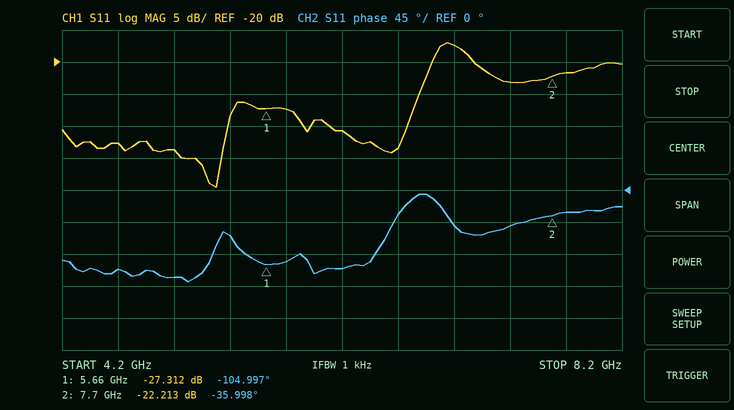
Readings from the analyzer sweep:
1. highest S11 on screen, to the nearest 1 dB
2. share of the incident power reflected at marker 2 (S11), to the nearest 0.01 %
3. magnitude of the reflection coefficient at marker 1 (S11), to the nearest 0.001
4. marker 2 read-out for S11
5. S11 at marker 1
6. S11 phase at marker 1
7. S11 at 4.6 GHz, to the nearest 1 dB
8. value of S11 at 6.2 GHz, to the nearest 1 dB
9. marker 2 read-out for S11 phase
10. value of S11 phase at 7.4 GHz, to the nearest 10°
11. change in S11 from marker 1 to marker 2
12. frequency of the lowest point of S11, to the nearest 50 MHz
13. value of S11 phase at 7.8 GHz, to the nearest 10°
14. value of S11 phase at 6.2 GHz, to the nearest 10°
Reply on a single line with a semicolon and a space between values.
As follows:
-17 dB; 0.60 %; 0.043; -22.213 dB; -27.312 dB; -104.997°; -33 dB; -31 dB; -35.998°; -50°; 5.099 dB; 5.30 GHz; -30°; -110°
